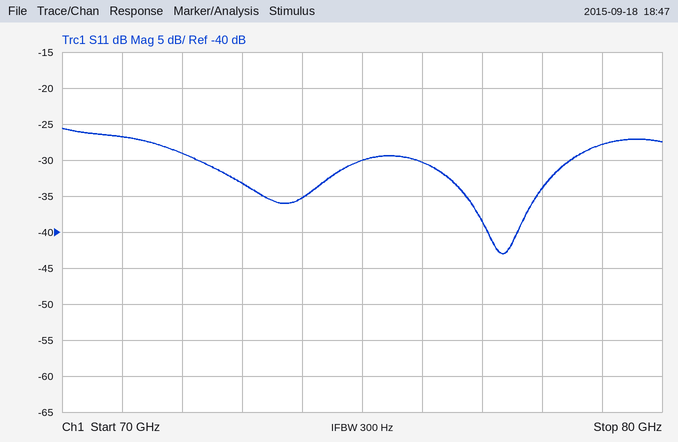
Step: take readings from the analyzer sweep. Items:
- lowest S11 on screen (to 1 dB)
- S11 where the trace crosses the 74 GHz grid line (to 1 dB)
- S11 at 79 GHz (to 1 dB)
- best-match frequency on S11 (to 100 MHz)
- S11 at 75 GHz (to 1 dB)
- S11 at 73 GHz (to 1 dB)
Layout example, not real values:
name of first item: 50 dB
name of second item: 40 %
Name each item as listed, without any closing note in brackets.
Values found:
lowest S11 on screen: -43 dB
S11 where the trace crosses the 74 GHz grid line: -35 dB
S11 at 79 GHz: -28 dB
best-match frequency on S11: 77.3 GHz
S11 at 75 GHz: -30 dB
S11 at 73 GHz: -33 dB
